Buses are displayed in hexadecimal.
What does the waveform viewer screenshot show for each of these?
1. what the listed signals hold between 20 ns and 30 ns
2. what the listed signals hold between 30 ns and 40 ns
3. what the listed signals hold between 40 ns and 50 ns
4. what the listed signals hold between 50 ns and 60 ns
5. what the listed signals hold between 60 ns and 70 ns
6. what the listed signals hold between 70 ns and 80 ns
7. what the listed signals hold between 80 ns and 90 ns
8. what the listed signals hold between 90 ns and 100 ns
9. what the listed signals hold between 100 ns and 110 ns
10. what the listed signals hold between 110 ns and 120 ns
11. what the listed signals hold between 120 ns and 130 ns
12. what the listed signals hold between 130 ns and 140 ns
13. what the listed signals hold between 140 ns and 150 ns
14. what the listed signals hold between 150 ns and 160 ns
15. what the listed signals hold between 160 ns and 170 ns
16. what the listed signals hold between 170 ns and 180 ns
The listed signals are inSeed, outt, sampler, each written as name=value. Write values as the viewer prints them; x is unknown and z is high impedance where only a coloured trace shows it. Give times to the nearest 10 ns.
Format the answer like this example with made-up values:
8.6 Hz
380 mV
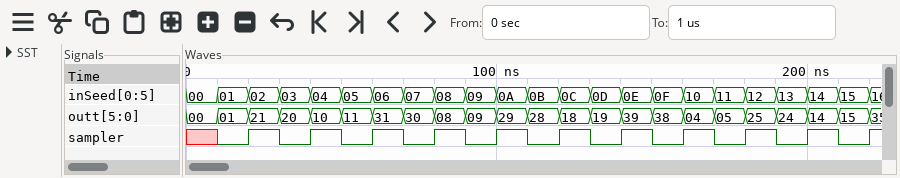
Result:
inSeed=02, outt=21, sampler=1
inSeed=03, outt=20, sampler=0
inSeed=04, outt=10, sampler=1
inSeed=05, outt=11, sampler=0
inSeed=06, outt=31, sampler=1
inSeed=07, outt=30, sampler=0
inSeed=08, outt=08, sampler=1
inSeed=09, outt=09, sampler=0
inSeed=0A, outt=29, sampler=1
inSeed=0B, outt=28, sampler=0
inSeed=0C, outt=18, sampler=1
inSeed=0D, outt=19, sampler=0
inSeed=0E, outt=39, sampler=1
inSeed=0F, outt=38, sampler=0
inSeed=10, outt=04, sampler=1
inSeed=11, outt=05, sampler=0
